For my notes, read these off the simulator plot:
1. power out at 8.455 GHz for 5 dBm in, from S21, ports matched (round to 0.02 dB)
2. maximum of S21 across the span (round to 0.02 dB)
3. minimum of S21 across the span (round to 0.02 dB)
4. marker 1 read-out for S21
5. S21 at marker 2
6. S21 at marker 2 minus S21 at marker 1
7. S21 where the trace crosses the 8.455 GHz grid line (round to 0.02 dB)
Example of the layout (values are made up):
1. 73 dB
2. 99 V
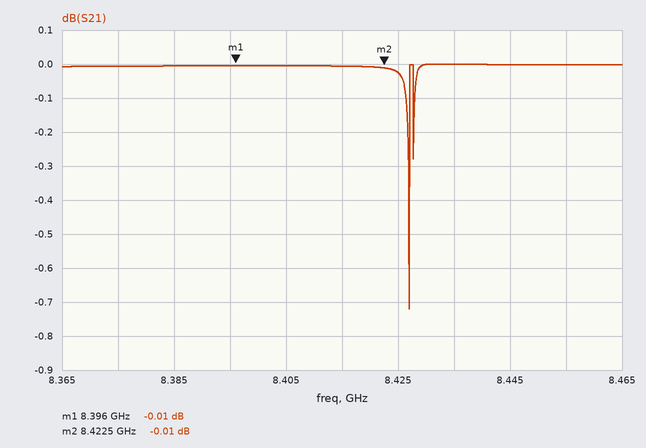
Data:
1. 5.00 dBm
2. 0.00 dB
3. -0.72 dB
4. -0.01 dB
5. -0.01 dB
6. 0.00 dB
7. 0.00 dB
